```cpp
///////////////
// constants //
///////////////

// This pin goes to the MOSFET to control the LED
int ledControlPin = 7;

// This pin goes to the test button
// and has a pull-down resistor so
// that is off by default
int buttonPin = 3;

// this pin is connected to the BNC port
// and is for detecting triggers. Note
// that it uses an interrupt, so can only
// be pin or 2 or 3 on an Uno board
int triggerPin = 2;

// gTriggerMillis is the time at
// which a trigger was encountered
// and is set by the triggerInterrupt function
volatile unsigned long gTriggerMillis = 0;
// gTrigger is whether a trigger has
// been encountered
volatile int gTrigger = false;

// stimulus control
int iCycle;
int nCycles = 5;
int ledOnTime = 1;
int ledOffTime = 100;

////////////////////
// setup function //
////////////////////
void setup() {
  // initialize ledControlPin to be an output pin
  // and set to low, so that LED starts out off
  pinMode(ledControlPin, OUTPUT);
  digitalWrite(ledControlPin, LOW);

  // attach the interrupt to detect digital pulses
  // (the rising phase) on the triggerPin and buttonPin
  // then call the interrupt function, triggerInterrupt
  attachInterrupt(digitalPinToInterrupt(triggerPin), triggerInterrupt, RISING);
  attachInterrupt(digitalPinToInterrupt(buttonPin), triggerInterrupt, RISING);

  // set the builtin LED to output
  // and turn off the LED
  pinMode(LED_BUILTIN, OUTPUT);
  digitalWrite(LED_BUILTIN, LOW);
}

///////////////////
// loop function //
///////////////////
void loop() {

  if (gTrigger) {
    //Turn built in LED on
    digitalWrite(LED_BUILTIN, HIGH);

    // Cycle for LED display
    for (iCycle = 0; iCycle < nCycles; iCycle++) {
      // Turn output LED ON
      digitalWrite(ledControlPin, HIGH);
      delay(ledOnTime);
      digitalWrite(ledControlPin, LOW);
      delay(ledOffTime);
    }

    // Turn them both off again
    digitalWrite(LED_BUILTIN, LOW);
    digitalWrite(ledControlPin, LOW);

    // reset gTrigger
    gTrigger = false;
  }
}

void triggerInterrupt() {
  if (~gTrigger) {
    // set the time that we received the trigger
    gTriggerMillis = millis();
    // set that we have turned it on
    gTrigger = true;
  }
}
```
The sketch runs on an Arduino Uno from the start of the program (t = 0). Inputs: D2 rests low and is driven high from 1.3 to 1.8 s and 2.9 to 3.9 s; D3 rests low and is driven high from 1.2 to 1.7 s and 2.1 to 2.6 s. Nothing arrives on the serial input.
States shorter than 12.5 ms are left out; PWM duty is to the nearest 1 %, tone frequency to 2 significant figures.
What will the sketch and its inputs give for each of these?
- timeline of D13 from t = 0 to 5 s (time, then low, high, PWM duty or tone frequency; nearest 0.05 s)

0 s low; 1.2 s high; 1.7 s low; 2.1 s high; 2.6 s low; 2.9 s high; 3.4 s low
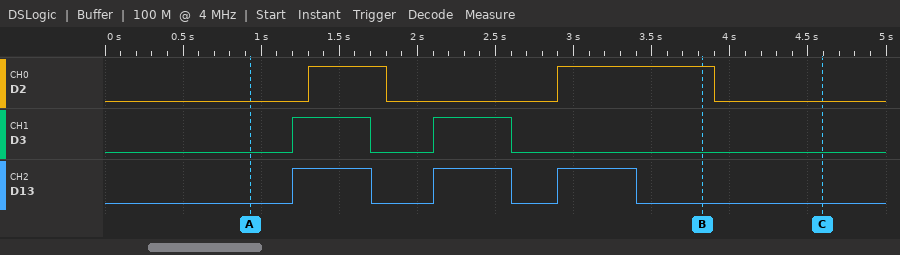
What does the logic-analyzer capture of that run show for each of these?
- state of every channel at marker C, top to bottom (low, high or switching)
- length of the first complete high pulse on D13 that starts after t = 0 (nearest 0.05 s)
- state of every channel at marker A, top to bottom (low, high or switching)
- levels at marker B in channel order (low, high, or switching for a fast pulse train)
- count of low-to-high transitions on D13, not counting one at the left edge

D2 low, D3 low, D13 low
0.50 s
D2 low, D3 low, D13 low
D2 high, D3 low, D13 low
3
